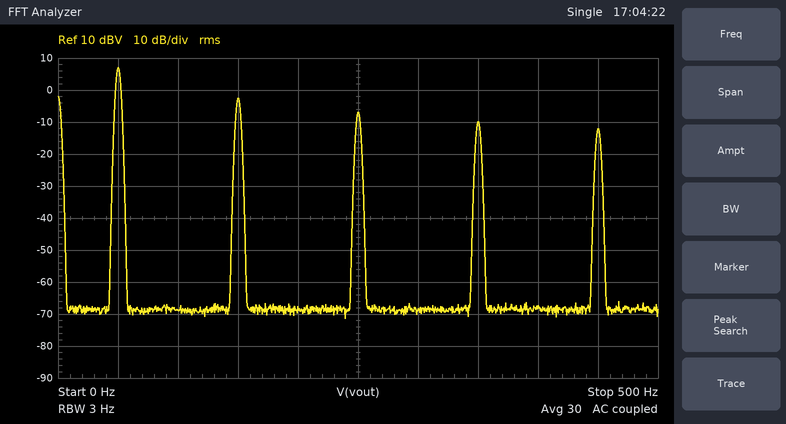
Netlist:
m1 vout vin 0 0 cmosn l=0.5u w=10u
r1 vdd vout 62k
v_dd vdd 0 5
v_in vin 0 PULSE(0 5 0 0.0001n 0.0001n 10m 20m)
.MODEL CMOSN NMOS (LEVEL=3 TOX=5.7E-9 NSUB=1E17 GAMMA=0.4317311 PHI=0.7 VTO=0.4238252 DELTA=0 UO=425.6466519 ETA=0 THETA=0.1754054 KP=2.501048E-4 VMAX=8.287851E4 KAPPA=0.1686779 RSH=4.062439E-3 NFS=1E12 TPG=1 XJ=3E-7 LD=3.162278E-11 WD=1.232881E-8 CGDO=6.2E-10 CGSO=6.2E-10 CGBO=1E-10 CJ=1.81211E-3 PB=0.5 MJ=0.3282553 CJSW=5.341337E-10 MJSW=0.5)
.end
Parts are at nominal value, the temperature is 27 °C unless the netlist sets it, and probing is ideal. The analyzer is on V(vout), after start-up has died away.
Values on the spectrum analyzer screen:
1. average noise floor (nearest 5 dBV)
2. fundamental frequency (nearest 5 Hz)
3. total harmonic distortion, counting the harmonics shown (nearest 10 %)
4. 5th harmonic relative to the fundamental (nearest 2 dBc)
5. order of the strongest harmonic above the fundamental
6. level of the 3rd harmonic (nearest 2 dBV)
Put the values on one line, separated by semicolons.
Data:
-70 dBV; 50 Hz; 40 %; -14 dBc; 3; -2 dBV
